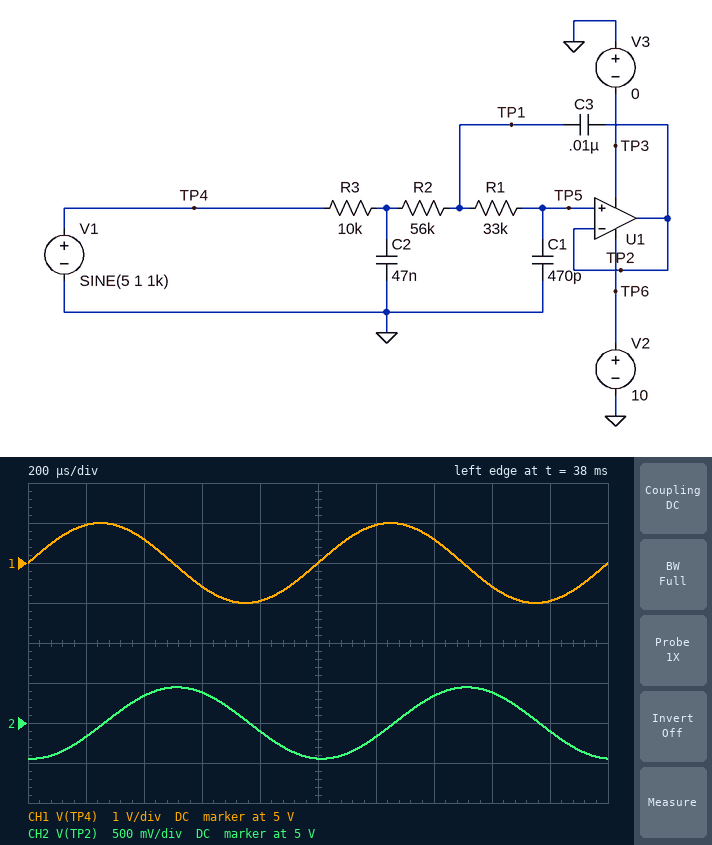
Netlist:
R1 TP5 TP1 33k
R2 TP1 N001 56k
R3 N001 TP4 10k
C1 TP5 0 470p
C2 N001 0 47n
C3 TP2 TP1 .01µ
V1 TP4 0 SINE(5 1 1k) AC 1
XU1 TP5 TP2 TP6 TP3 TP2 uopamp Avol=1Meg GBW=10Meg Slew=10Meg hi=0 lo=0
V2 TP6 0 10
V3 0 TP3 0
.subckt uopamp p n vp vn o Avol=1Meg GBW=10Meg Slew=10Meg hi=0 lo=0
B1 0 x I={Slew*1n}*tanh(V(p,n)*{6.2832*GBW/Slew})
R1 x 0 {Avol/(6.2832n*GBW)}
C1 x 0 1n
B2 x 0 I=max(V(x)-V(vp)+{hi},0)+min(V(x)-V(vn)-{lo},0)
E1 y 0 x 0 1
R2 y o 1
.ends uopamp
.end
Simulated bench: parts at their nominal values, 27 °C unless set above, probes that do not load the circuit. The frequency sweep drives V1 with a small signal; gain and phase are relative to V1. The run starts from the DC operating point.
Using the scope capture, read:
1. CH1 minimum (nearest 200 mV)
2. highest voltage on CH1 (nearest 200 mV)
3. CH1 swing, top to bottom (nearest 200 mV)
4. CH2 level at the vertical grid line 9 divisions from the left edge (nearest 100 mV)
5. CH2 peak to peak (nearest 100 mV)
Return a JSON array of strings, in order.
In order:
["4.0 V", "6.0 V", "2.0 V", "4.9 V", "900 mV"]
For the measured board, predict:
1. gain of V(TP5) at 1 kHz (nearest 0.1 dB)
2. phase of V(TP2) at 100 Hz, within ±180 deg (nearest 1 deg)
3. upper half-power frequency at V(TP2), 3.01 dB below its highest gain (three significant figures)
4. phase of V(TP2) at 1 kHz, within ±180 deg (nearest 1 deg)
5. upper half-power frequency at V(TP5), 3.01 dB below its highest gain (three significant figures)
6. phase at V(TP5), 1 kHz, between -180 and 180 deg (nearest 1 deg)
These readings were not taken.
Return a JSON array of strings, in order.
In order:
["-7.0 dB", "-18 deg", "365 Hz", "-95 deg", "365 Hz", "-95 deg"]
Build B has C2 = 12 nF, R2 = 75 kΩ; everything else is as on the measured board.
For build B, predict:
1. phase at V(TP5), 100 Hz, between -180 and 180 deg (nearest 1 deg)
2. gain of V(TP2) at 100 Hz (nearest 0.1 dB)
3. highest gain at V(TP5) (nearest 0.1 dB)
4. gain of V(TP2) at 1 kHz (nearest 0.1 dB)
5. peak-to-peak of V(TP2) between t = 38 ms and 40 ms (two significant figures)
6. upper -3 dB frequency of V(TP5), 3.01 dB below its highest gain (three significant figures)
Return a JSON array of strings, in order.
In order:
["-6 deg", "0 dB", "2.8 dB", "2.0 dB", "2.5 V", "1.61 kHz"]
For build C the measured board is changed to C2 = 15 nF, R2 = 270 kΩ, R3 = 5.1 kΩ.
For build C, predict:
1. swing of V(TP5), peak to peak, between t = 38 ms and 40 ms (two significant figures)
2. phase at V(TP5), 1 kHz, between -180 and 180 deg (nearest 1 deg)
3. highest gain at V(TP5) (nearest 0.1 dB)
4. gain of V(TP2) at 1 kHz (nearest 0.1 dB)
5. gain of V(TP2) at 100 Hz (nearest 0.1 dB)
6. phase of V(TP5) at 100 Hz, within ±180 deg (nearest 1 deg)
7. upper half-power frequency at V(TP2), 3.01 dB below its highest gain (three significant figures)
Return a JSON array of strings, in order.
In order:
["1.6 V", "-152 deg", "3.2 dB", "-2.0 dB", "0.1 dB", "-8 deg", "900 Hz"]
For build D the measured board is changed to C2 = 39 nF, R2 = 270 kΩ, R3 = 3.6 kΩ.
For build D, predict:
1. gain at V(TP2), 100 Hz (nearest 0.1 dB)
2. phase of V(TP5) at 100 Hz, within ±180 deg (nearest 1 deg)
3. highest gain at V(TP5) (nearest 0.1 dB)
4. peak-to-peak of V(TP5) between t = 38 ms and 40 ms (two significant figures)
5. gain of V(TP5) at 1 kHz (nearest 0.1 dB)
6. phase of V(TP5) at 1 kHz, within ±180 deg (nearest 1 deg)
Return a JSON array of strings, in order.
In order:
["0.1 dB", "-10 deg", "2.4 dB", "1.3 V", "-3.5 dB", "-167 deg"]
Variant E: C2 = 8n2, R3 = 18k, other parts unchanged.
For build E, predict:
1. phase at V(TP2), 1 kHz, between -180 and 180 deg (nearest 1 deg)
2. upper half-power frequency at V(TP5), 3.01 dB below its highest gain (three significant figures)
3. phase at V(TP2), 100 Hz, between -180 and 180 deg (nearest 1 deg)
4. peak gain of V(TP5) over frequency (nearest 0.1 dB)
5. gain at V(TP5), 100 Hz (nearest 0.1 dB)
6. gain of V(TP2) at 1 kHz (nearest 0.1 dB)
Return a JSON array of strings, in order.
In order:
["-72 deg", "1.80 kHz", "-7 deg", "0.6 dB", "0 dB", "0.2 dB"]
